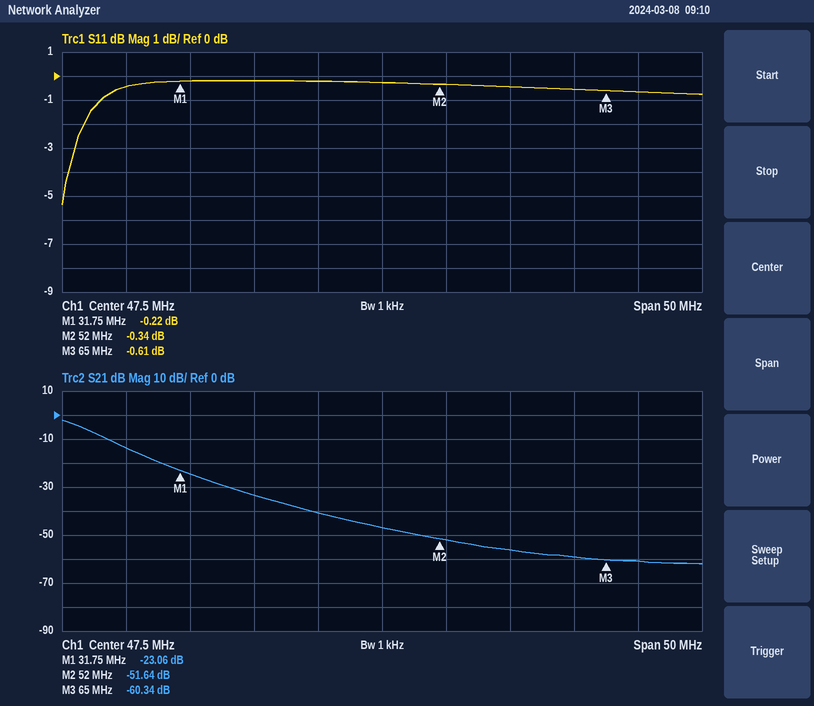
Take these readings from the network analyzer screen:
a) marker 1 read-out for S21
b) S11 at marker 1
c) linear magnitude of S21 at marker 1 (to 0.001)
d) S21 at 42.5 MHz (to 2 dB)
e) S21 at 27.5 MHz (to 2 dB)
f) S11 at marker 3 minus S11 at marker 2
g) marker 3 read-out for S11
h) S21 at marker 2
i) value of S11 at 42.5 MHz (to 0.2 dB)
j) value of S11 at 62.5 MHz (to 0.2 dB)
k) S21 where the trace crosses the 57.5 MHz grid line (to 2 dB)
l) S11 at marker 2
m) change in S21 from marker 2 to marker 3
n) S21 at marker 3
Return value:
-23.06 dB
-0.22 dB
0.070
-40 dB
-14 dB
-0.27 dB
-0.61 dB
-51.64 dB
-0.2 dB
-0.6 dB
-56 dB
-0.34 dB
-8.70 dB
-60.34 dB
